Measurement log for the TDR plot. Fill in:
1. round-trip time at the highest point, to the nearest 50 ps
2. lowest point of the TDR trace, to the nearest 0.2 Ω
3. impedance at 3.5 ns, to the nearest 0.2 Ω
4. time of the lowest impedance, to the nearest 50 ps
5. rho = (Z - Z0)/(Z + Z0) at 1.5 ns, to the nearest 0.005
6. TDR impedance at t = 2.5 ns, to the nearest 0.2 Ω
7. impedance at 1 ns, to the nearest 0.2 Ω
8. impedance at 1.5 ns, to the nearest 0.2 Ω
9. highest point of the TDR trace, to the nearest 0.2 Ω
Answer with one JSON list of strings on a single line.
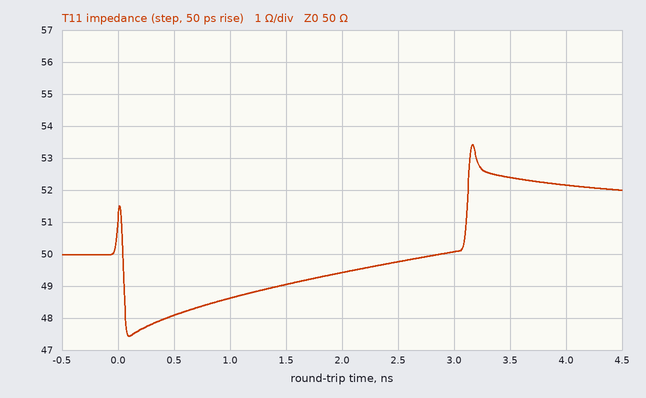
["3.15 ns", "47.4 Ω", "52.4 Ω", "100 ps", "-0.010", "49.8 Ω", "48.6 Ω", "49.0 Ω", "53.4 Ω"]
